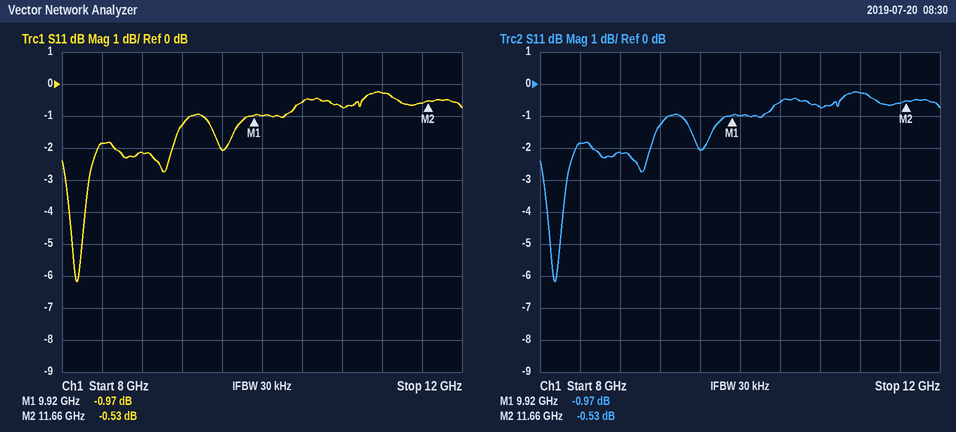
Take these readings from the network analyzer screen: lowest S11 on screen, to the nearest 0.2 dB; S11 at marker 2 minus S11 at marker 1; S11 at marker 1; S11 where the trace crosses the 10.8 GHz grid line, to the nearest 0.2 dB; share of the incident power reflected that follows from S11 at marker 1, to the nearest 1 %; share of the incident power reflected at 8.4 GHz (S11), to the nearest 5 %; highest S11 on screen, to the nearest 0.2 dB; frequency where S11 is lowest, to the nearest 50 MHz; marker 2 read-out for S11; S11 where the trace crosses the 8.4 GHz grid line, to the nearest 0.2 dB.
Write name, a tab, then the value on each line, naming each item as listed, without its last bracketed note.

lowest S11 on screen, to the nearest 0.2 dB	-6.2 dB
S11 at marker 2 minus S11 at marker 1	0.44 dB
S11 at marker 1	-0.97 dB
S11 where the trace crosses the 10.8 GHz grid line, to the nearest 0.2 dB	-0.8 dB
share of the incident power reflected that follows from S11 at marker 1, to the nearest 1 %	80 %
share of the incident power reflected at 8.4 GHz (S11), to the nearest 5 %	65 %
highest S11 on screen, to the nearest 0.2 dB	-0.2 dB
frequency where S11 is lowest, to the nearest 50 MHz	8.15 GHz
marker 2 read-out for S11	-0.53 dB
S11 where the trace crosses the 8.4 GHz grid line, to the nearest 0.2 dB	-1.8 dB
